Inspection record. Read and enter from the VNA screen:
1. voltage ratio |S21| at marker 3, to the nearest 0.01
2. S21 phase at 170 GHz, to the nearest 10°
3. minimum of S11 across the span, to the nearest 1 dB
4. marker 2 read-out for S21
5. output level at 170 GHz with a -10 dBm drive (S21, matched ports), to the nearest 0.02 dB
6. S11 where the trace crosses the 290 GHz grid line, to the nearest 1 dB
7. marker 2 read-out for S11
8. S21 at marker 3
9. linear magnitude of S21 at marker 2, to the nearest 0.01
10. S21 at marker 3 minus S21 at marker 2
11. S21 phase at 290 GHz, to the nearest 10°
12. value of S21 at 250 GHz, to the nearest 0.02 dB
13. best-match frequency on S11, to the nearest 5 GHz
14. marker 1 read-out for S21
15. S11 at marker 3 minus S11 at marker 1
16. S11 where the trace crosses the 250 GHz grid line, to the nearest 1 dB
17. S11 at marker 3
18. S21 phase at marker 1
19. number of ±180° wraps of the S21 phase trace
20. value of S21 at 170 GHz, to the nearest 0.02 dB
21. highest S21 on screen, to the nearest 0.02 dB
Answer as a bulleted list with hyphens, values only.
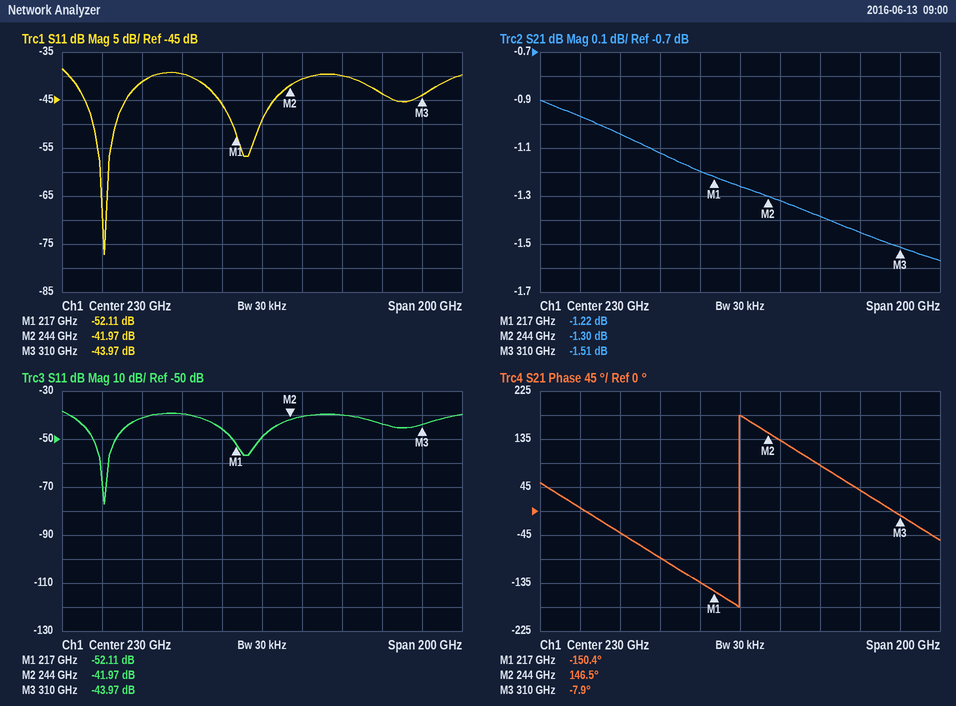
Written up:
- 0.84
- -40°
- -77 dB
- -1.30 dB
- -11.04 dBm
- -44 dB
- -41.97 dB
- -1.51 dB
- 0.86
- -0.21 dB
- 40°
- -1.32 dB
- 150 GHz
- -1.22 dB
- 8.14 dB
- -41 dB
- -43.97 dB
- -150.4°
- 1
- -1.04 dB
- -0.90 dB
